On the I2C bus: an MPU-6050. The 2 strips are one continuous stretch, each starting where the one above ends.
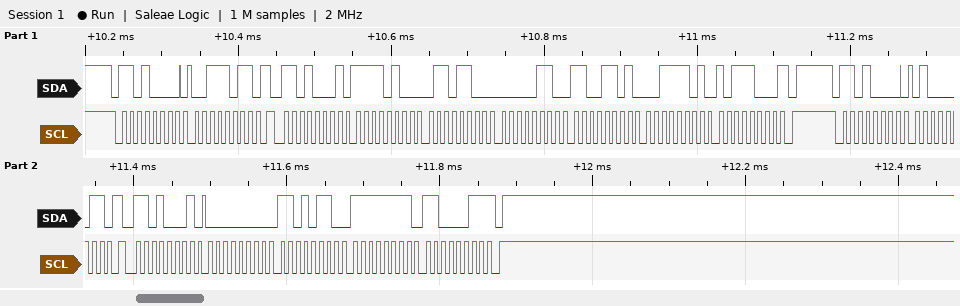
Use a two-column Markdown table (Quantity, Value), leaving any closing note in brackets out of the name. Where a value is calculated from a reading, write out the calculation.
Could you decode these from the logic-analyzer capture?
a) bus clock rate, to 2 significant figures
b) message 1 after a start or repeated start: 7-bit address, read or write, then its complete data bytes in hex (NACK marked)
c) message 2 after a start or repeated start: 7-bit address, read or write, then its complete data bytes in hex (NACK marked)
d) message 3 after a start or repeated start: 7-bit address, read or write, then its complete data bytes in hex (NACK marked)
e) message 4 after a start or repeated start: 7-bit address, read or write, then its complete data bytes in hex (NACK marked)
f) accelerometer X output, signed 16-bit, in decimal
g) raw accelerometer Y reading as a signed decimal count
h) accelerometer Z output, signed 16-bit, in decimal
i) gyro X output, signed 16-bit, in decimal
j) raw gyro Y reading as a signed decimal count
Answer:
| Quantity | Value |
|---|---|
| bus clock rate, to 2 significant figures | 100 kHz |
| message 1 after a start or repeated start: 7-bit address, read or write, then its complete data bytes in hex | 0x68 write: 3B |
| message 2 after a start or repeated start: 7-bit address, read or write, then its complete data bytes in hex | 0x68 read: F4 6C 06 CD 3D B8 NACK |
| message 3 after a start or repeated start: 7-bit address, read or write, then its complete data bytes in hex | 0x68 write: 43 |
| message 4 after a start or repeated start: 7-bit address, read or write, then its complete data bytes in hex | 0x68 read: 00 D6 FF C3 NACK |
| accelerometer X output, signed 16-bit, in decimal | 0xF46C = -2964 |
| raw accelerometer Y reading as a signed decimal count | 0x06CD = 1741 |
| accelerometer Z output, signed 16-bit, in decimal | 0x3DB8 = 15800 |
| gyro X output, signed 16-bit, in decimal | 0x00D6 = 214 |
| raw gyro Y reading as a signed decimal count | 0xFFC3 = -61 |
